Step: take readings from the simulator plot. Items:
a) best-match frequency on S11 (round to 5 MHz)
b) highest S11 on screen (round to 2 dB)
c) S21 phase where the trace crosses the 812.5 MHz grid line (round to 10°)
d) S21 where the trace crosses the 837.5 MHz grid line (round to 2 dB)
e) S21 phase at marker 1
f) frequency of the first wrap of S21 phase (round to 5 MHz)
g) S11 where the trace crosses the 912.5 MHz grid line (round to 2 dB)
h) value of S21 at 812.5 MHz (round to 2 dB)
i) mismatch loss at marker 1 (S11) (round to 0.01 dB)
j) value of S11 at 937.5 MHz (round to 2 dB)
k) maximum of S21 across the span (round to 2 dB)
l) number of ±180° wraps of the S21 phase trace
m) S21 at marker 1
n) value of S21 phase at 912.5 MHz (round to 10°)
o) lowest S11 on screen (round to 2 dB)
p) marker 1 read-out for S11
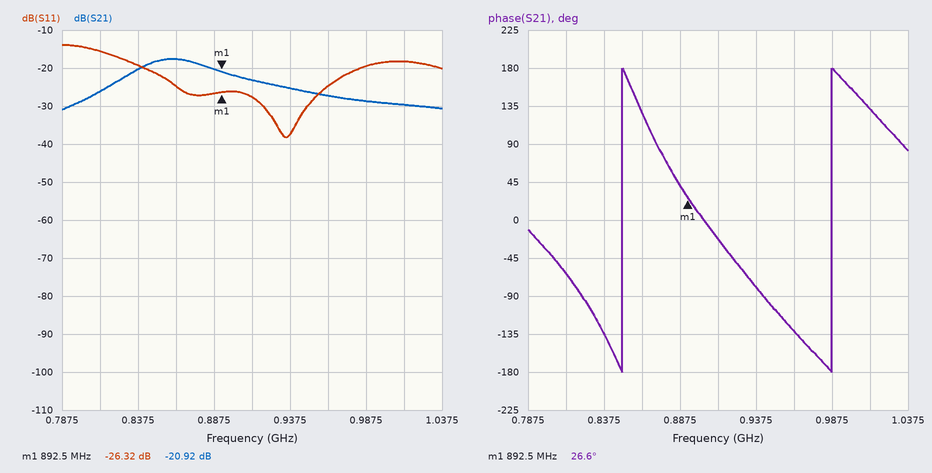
935 MHz
-14 dB
-60°
-20 dB
26.6°
850 MHz
-28 dB
-26 dB
0.01 dB
-38 dB
-18 dB
2
-20.92 dB
-20°
-38 dB
-26.32 dB
